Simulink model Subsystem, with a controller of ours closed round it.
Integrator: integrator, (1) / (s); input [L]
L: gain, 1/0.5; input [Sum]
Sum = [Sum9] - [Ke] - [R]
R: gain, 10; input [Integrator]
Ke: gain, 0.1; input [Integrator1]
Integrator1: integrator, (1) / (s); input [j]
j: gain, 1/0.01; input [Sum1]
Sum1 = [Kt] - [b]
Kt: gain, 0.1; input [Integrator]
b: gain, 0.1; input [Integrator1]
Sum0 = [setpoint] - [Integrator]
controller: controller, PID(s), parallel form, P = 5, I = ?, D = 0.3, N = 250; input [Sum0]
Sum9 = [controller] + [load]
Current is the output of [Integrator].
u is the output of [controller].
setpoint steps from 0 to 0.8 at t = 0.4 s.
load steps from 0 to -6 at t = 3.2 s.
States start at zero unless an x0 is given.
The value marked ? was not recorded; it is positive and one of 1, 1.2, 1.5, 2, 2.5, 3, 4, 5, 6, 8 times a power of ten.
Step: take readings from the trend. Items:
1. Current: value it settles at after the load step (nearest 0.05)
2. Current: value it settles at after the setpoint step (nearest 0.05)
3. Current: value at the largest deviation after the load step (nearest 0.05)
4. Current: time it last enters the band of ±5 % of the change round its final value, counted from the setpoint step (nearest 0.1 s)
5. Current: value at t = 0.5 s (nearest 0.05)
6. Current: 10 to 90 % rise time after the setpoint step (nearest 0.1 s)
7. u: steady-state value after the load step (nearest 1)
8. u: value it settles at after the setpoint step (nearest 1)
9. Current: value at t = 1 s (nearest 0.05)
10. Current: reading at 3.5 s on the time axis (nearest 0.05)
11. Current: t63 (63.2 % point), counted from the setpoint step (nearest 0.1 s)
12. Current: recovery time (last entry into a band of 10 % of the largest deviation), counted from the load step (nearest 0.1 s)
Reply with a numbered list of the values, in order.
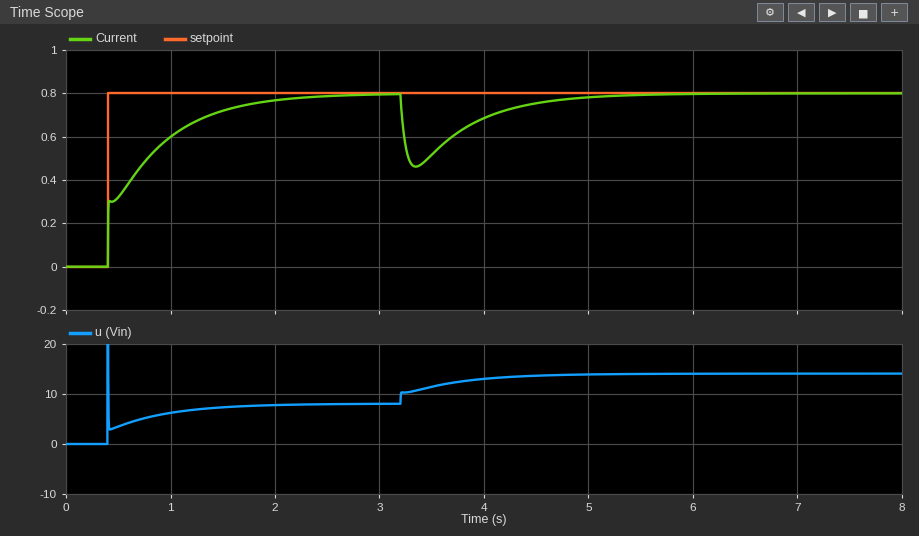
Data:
1. 0.80
2. 0.80
3. 0.45
4. 1.5 s
5. 0.30
6. 1.1 s
7. 14
8. 8
9. 0.60
10. 0.50
11. 0.4 s
12. 1.5 s
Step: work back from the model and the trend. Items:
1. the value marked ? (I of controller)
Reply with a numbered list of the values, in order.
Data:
1. 25
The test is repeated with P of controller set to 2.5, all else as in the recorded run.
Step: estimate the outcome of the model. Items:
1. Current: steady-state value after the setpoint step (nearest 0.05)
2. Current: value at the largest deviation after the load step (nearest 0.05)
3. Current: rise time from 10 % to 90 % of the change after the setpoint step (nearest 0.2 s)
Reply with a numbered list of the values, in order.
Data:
1. 0.80
2. 0.40
3. 1.0 s
